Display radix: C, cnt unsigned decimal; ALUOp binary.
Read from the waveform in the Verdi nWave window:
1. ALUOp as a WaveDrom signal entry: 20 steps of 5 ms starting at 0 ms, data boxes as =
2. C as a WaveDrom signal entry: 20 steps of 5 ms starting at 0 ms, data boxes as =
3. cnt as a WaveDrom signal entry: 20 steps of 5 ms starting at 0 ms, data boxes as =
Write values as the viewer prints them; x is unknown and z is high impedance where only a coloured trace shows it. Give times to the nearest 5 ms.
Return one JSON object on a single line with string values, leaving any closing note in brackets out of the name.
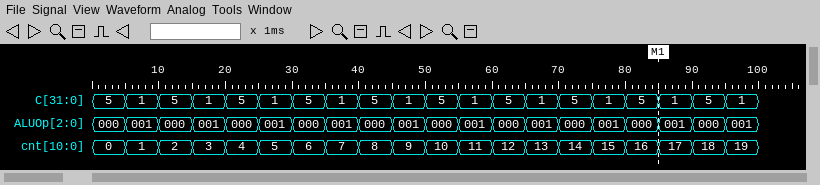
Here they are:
{"ALUOp as a WaveDrom signal entry: 20 steps of 5 ms starting at 0 ms, data boxes as =": "{name: 'ALUOp', wave: '====================', data: '000 001 000 001 000 001 000 001 000 001 000 001 000 001 000 001 000 001 000 001'}", "C as a WaveDrom signal entry: 20 steps of 5 ms starting at 0 ms, data boxes as =": "{name: 'C', wave: '====================', data: '5 1 5 1 5 1 5 1 5 1 5 1 5 1 5 1 5 1 5 1'}", "cnt as a WaveDrom signal entry: 20 steps of 5 ms starting at 0 ms, data boxes as =": "{name: 'cnt', wave: '====================', data: '0 1 2 3 4 5 6 7 8 9 10 11 12 13 14 15 16 17 18 19'}"}
